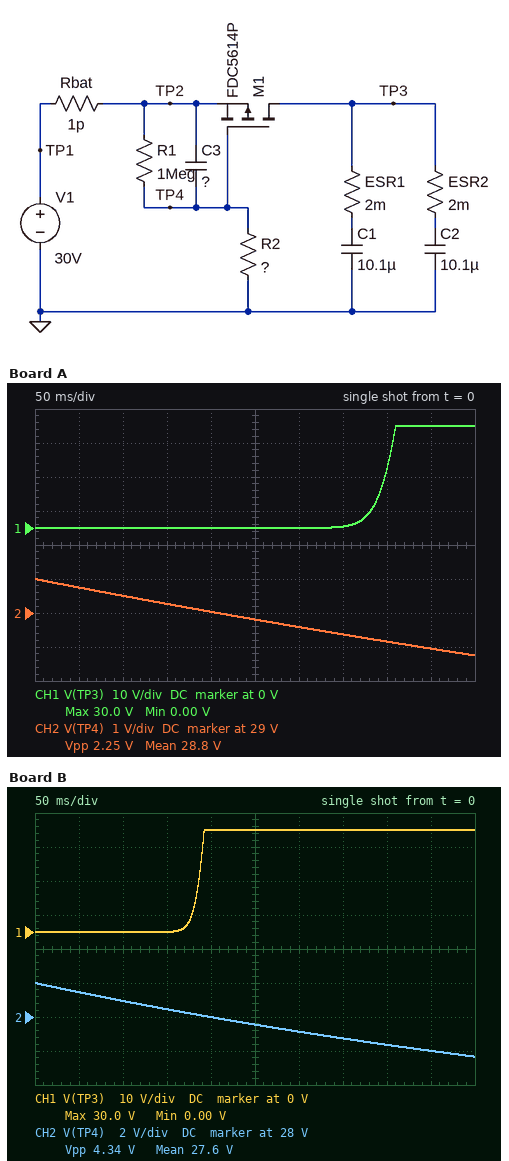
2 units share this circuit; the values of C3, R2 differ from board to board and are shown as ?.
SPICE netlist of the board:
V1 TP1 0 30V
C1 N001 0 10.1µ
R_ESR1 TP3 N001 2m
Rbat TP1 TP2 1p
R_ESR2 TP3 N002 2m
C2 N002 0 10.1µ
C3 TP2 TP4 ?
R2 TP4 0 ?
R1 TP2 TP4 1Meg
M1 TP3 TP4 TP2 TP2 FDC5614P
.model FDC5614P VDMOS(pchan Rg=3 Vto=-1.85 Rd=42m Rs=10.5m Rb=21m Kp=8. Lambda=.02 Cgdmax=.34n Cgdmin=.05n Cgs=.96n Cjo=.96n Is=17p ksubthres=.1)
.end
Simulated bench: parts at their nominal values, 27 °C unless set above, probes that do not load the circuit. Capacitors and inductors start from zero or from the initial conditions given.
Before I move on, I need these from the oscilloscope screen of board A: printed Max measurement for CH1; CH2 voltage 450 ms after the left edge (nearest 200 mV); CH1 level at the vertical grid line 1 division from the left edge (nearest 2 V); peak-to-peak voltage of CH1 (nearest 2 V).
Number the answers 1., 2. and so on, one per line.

1. 30.0 V
2. 28.0 V
3. 0 V
4. 30 V
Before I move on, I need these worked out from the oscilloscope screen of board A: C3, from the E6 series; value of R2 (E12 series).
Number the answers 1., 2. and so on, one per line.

1. 3.3 µF
2. 1.8 MΩ
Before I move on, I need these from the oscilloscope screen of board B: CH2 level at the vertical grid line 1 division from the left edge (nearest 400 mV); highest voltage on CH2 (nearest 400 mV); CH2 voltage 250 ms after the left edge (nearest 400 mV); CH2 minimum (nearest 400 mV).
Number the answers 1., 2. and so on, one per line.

1. 29.6 V
2. 30.0 V
3. 27.6 V
4. 25.6 V
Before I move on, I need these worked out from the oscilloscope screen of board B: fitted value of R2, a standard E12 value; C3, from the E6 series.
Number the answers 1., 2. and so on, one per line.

1. 1.8 MΩ
2. 1.5 µF
